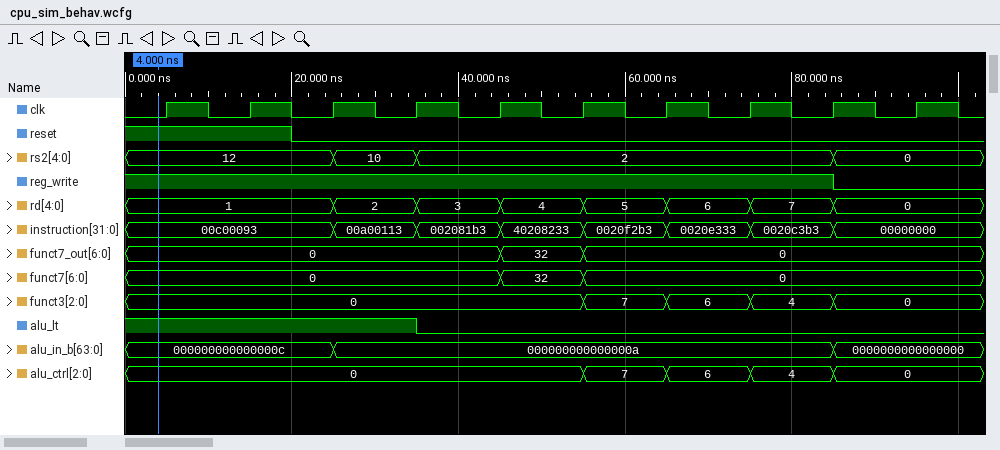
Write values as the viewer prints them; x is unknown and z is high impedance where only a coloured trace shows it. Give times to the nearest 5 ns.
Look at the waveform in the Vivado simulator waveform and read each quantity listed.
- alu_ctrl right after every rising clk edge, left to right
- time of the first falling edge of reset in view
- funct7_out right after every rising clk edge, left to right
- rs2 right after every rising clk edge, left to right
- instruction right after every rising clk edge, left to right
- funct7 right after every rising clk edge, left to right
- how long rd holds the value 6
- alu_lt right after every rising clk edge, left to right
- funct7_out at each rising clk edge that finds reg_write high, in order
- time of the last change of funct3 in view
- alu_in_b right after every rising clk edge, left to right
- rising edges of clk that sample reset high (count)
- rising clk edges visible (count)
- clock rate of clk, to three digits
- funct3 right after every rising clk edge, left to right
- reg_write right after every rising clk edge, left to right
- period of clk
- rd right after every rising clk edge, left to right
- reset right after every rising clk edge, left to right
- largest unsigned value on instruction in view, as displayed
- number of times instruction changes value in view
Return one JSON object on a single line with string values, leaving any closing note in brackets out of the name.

{"alu_ctrl right after every rising clk edge, left to right": "0, 0, 0, 0, 0, 7, 6, 4, 0, 0", "time of the first falling edge of reset in view": "20 ns", "funct7_out right after every rising clk edge, left to right": "0, 0, 0, 0, 32, 0, 0, 0, 0, 0", "rs2 right after every rising clk edge, left to right": "12, 12, 10, 2, 2, 2, 2, 2, 0, 0", "instruction right after every rising clk edge, left to right": "00c00093, 00c00093, 00a00113, 002081b3, 40208233, 0020f2b3, 0020e333, 0020c3b3, 00000000, 00000000", "funct7 right after every rising clk edge, left to right": "0, 0, 0, 0, 32, 0, 0, 0, 0, 0", "how long rd holds the value 6": "10 ns", "alu_lt right after every rising clk edge, left to right": "1 1 1 0 0 0 0 0 0 0", "funct7_out at each rising clk edge that finds reg_write high, in order": "0, 0, 0, 0, 0, 32, 0, 0, 0", "time of the last change of funct3 in view": "85 ns", "alu_in_b right after every rising clk edge, left to right": "000000000000000c, 000000000000000c, 000000000000000a, 000000000000000a, 000000000000000a, 000000000000000a, 000000000000000a, 000000000000000a, 0000000000000000, 0000000000000000", "rising edges of clk that sample reset high": "2", "rising clk edges visible": "10", "clock rate of clk, to three digits": "100 MHz", "funct3 right after every rising clk edge, left to right": "0, 0, 0, 0, 0, 7, 6, 4, 0, 0", "reg_write right after every rising clk edge, left to right": "1 1 1 1 1 1 1 1 0 0", "period of clk": "10 ns", "rd right after every rising clk edge, left to right": "1, 1, 2, 3, 4, 5, 6, 7, 0, 0", "reset right after every rising clk edge, left to right": "1 1 0 0 0 0 0 0 0 0", "largest unsigned value on instruction in view, as displayed": "40208233", "number of times instruction changes value in view": "7"}
